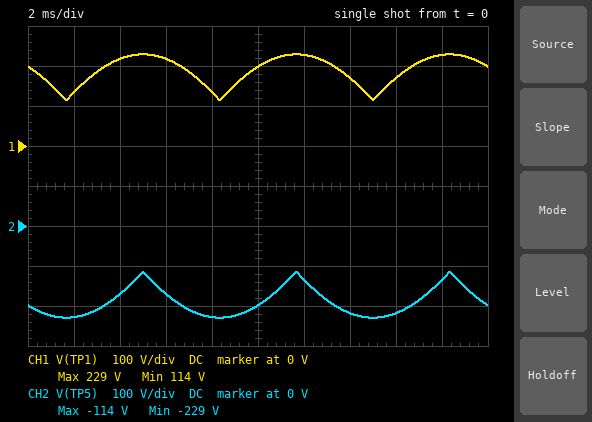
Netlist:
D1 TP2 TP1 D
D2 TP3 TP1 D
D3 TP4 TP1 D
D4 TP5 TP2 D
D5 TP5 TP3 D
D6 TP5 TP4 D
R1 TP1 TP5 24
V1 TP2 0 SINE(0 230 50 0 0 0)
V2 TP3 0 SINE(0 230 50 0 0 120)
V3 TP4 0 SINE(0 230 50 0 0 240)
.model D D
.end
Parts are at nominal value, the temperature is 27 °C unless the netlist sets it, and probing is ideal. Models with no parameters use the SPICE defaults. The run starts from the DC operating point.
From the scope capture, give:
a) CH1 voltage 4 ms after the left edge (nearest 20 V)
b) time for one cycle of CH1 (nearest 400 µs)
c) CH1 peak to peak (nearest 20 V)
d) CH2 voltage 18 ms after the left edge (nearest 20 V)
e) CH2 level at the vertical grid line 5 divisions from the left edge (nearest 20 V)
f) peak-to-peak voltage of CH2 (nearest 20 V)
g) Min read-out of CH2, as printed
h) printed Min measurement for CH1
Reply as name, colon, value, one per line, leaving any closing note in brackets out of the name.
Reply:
CH1 voltage 4 ms after the left edge: 220 V
time for one cycle of CH1: 6.8 ms
CH1 peak to peak: 120 V
CH2 voltage 18 ms after the left edge: -140 V
CH2 level at the vertical grid line 5 divisions from the left edge: -200 V
peak-to-peak voltage of CH2: 120 V
Min read-out of CH2, as printed: -229 V
printed Min measurement for CH1: 114 V
